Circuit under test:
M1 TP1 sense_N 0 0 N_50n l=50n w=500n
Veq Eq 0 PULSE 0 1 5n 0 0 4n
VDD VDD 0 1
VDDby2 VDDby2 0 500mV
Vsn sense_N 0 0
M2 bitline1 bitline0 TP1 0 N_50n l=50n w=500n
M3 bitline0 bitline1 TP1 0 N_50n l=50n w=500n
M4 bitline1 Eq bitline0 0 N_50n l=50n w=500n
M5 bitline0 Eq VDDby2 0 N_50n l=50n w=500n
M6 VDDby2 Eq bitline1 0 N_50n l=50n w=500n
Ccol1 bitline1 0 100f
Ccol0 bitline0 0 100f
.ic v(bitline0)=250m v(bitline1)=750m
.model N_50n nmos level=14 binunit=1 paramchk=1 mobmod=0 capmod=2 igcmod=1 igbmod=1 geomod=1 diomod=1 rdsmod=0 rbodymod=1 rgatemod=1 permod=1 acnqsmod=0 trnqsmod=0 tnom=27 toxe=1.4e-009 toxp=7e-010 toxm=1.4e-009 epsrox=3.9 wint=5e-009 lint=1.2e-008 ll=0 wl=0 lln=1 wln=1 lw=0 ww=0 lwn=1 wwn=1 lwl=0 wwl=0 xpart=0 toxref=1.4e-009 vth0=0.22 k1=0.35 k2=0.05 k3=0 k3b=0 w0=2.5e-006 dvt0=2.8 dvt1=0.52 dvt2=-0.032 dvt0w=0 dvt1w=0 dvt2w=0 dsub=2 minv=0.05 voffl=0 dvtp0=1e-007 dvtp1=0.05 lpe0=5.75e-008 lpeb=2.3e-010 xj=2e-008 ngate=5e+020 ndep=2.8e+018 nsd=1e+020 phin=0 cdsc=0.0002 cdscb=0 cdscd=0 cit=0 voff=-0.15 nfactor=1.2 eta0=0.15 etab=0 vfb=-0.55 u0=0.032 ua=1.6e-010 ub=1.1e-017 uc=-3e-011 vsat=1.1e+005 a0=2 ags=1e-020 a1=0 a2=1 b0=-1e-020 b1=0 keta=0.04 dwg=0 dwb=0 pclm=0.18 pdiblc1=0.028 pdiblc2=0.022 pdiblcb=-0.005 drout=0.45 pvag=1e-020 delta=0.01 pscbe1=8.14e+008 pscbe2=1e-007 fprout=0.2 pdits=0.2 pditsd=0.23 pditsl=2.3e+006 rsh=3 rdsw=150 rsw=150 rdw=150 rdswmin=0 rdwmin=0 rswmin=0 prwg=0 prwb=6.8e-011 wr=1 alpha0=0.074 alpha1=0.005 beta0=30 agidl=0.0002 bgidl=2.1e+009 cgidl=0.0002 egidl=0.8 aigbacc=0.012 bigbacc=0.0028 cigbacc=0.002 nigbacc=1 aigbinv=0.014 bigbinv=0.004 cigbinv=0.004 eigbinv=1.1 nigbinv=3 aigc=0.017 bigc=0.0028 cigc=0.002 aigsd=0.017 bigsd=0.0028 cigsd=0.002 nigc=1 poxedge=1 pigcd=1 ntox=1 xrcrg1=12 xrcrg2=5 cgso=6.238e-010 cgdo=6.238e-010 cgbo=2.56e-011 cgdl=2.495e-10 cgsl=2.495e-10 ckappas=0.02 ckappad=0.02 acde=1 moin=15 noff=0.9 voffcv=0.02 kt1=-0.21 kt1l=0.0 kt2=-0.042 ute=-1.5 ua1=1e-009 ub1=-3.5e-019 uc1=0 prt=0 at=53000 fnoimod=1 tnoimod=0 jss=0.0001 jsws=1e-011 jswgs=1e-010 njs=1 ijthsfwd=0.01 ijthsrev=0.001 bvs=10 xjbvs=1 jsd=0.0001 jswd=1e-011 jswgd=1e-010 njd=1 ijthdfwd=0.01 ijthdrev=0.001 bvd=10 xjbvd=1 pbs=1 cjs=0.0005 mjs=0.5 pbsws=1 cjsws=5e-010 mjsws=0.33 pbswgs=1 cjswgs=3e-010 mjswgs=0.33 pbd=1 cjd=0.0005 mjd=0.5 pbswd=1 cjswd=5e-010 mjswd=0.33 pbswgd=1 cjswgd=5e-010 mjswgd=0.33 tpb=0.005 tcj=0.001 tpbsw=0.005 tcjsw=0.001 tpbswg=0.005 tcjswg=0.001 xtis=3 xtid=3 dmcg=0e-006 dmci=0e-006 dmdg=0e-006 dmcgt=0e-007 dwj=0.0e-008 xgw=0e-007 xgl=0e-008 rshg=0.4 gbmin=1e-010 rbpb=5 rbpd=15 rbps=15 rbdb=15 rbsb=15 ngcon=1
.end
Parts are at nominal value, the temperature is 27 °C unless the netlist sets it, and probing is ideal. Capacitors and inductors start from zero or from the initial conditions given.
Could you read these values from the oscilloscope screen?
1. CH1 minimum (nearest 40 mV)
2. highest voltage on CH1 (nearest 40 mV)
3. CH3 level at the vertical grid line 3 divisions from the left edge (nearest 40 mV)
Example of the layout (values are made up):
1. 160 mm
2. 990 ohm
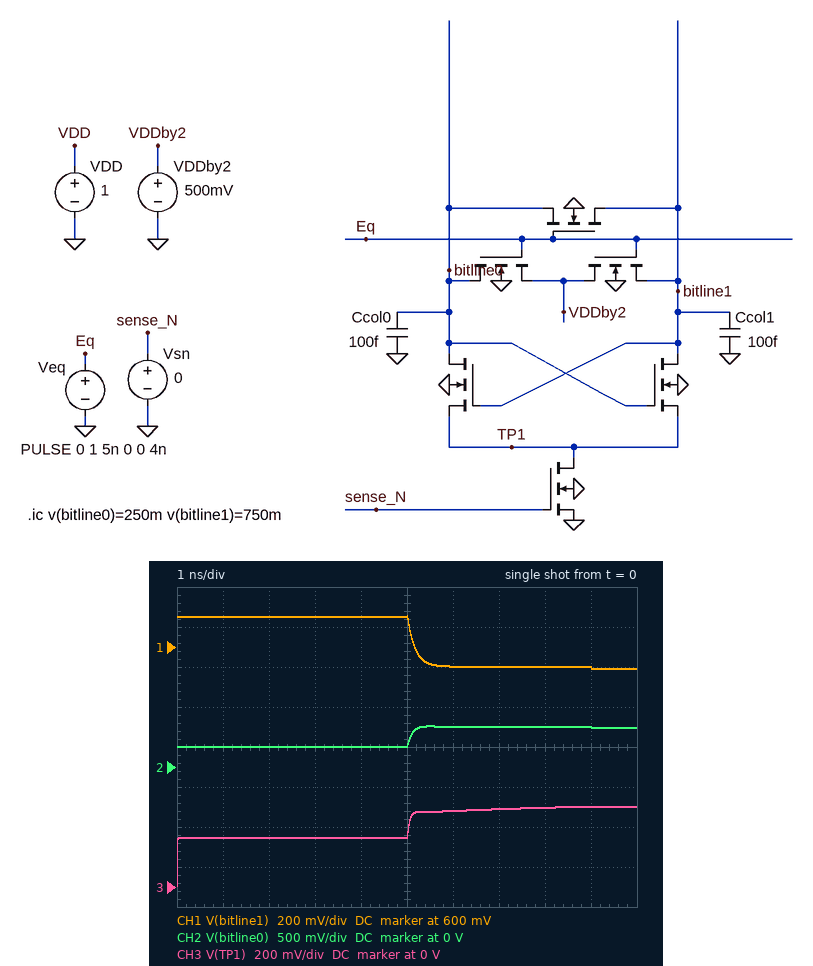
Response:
1. 480 mV
2. 760 mV
3. 240 mV
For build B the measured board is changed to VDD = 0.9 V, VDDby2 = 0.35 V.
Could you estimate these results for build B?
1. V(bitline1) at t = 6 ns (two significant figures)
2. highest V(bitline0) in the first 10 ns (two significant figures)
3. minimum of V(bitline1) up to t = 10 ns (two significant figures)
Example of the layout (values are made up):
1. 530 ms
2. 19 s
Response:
1. 350 mV
2. 400 mV
3. 340 mV
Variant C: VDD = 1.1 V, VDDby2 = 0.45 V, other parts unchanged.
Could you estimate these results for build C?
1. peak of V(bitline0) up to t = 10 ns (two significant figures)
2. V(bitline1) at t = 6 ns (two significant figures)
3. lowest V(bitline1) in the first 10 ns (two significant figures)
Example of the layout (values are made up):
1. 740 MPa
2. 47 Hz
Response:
1. 470 mV
2. 450 mV
3. 440 mV
